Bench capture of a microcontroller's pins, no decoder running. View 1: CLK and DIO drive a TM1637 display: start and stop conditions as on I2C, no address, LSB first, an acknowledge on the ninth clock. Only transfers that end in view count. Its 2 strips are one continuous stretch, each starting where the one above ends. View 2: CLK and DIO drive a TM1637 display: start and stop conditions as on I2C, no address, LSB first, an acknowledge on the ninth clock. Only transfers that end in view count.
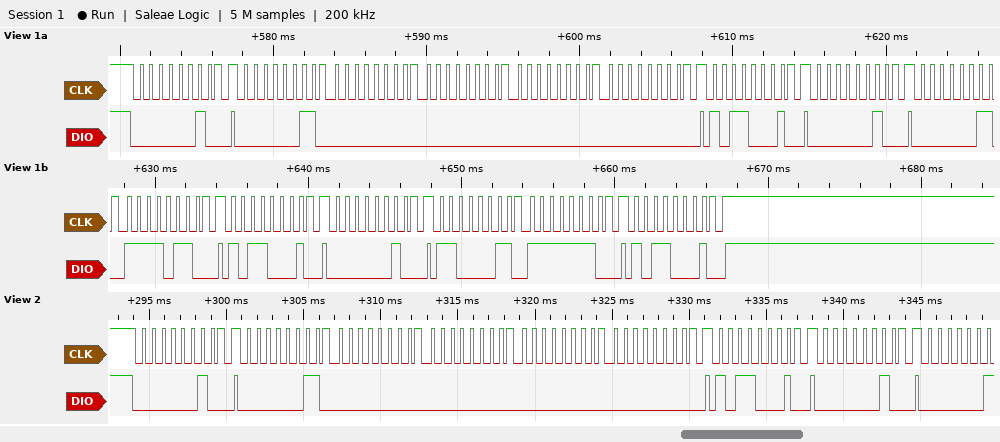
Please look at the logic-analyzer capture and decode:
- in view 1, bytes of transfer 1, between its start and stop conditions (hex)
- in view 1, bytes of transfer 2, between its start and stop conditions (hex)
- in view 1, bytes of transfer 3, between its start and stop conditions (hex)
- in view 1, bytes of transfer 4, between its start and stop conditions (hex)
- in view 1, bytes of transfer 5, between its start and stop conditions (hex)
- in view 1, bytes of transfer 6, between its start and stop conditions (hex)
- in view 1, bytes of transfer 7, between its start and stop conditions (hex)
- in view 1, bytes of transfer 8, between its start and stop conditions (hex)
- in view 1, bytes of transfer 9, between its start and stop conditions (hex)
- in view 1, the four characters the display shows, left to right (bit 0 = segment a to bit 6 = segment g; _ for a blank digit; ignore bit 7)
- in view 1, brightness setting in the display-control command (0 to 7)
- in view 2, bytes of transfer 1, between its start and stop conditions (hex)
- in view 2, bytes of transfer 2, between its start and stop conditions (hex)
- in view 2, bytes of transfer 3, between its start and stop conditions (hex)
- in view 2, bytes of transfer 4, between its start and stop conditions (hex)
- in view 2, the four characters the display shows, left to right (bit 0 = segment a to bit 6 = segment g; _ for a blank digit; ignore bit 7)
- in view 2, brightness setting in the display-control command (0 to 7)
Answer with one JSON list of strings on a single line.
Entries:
["40", "C0 00 00 00 00", "8D", "40", "C0 6F", "8D", "40", "C3 7F", "8D", "9__8", "5", "40", "C0 00 00 00 00", "8D", "40", "____", "5"]
